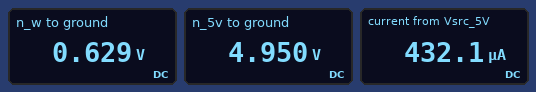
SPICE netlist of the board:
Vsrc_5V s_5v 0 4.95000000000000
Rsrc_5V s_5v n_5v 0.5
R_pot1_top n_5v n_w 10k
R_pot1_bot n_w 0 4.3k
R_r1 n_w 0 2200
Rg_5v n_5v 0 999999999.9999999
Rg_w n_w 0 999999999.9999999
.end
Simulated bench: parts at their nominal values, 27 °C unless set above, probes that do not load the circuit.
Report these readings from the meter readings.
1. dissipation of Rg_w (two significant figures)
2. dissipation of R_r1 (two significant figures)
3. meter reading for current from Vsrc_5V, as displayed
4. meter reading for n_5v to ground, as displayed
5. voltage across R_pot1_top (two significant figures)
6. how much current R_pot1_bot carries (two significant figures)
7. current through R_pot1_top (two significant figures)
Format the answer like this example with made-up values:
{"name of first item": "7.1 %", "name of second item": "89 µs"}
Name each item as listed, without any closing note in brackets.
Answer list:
{"dissipation of Rg_w": "400 pW", "dissipation of R_r1": "180 µW", "meter reading for current from Vsrc_5V, as displayed": "432.1 µA", "meter reading for n_5v to ground, as displayed": "4.950 V", "voltage across R_pot1_top": "4.3 V", "how much current R_pot1_bot carries": "150 µA", "current through R_pot1_top": "430 µA"}
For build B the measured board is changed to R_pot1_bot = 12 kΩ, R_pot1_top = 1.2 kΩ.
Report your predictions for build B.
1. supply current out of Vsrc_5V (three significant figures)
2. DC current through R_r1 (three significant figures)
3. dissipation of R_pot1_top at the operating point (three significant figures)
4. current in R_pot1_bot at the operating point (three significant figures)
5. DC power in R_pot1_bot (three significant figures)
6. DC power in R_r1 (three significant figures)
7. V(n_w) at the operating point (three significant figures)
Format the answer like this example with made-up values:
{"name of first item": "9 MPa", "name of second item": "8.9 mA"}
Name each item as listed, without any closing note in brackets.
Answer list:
{"supply current out of Vsrc_5V": "1.62 mA", "DC current through R_r1": "1.37 mA", "dissipation of R_pot1_top at the operating point": "3.14 mW", "current in R_pot1_bot at the operating point": "251 µA", "DC power in R_pot1_bot": "754 µW", "DC power in R_r1": "4.11 mW", "V(n_w) at the operating point": "3.01 V"}
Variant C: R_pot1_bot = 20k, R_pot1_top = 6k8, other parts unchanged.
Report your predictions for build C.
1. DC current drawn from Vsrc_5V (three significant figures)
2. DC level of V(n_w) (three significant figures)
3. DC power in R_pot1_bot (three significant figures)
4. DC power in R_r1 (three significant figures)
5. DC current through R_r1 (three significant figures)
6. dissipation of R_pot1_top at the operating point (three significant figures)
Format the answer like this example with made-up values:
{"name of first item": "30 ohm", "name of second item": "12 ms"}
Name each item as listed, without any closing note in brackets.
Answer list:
{"DC current drawn from Vsrc_5V": "564 µA", "DC level of V(n_w)": "1.12 V", "DC power in R_pot1_bot": "62.4 µW", "DC power in R_r1": "567 µW", "DC current through R_r1": "508 µA", "dissipation of R_pot1_top at the operating point": "2.16 mW"}
